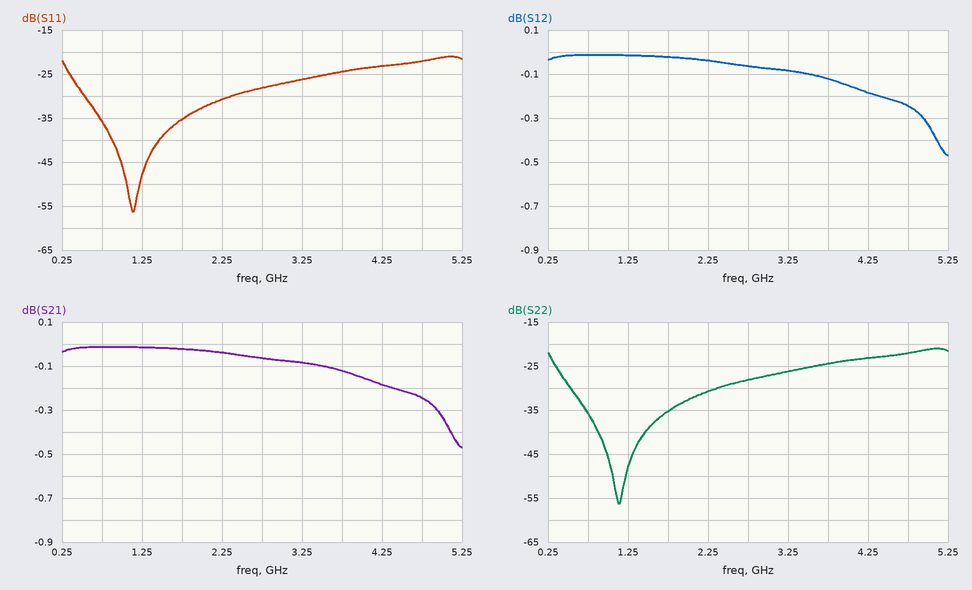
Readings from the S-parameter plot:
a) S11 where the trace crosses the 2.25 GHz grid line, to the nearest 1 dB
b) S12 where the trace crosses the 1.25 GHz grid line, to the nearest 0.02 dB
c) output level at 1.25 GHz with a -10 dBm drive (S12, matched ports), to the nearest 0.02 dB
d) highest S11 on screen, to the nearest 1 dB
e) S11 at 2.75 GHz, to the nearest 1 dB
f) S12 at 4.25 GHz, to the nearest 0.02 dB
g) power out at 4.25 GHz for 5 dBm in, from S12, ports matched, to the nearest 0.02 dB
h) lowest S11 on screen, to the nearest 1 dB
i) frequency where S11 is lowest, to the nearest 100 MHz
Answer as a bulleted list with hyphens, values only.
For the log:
- -31 dB
- -0.02 dB
- -10.02 dBm
- -21 dB
- -28 dB
- -0.18 dB
- 4.82 dBm
- -56 dB
- 1.1 GHz
